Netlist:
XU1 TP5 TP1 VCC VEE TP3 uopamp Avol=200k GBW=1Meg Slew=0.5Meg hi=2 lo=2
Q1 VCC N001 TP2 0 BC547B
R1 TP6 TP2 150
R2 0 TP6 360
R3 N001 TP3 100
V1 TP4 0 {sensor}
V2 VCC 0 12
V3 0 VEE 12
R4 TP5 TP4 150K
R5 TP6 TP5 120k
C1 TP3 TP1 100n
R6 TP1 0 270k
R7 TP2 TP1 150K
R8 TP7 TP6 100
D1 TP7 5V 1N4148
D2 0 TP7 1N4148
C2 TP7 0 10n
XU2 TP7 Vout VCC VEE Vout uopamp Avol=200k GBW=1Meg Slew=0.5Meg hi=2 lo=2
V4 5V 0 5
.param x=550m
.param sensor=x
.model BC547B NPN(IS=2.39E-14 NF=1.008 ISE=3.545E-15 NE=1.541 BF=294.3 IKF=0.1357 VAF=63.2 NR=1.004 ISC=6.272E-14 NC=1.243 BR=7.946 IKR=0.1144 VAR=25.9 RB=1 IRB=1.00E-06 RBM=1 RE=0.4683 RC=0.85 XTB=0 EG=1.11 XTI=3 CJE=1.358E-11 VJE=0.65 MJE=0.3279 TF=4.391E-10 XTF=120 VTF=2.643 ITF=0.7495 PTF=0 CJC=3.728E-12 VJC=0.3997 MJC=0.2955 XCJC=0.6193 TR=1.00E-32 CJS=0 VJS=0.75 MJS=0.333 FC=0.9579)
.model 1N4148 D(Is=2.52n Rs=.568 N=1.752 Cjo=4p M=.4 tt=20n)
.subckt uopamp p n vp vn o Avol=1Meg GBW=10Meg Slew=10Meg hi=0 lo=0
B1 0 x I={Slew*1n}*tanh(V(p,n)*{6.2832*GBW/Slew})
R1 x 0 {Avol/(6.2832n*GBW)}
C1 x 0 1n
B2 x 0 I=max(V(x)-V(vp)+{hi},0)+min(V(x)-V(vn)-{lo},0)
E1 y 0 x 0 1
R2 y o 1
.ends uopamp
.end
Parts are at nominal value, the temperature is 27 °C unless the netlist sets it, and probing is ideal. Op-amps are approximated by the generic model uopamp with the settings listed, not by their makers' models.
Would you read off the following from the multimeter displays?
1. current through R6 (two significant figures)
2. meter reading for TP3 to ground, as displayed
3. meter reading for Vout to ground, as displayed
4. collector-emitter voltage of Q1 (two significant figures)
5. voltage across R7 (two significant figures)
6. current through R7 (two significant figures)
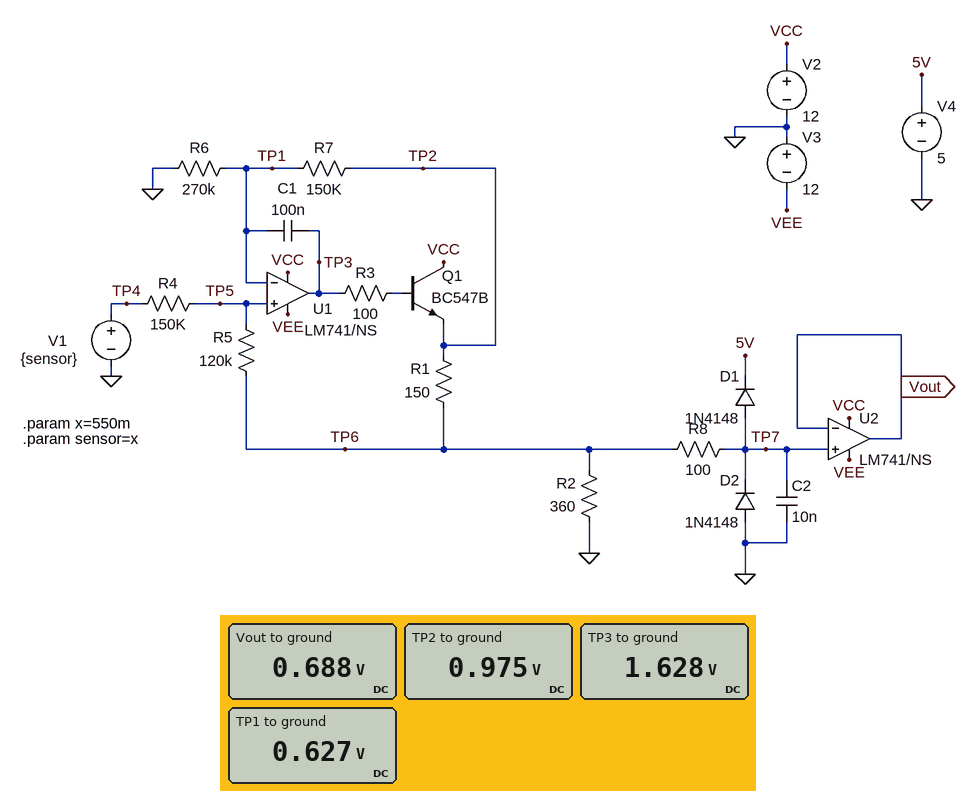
2.3 µA
1.628 V
0.688 V
11 V
350 mV
2.3 µA
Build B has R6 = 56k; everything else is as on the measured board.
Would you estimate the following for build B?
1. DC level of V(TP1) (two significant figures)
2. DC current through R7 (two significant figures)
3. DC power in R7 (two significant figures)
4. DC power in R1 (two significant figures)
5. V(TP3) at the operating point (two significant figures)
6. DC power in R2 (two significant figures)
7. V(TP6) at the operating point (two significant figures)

2.5 V
45 µA
300 µW
67 mW
10 V
100 mW
6.1 V
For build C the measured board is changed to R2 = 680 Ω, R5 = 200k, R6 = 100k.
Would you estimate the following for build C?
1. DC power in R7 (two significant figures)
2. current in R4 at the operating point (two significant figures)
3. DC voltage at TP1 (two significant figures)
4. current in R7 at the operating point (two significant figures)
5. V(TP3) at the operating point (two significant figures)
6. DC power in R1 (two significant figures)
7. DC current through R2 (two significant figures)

99 µW
13 µA
2.6 V
26 µA
7.1 V
9.0 mW
7.7 mA
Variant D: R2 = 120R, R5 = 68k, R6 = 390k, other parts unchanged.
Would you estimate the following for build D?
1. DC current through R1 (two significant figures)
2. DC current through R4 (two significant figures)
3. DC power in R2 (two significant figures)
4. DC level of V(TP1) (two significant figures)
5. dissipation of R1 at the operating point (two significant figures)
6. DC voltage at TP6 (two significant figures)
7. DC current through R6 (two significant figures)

1.5 mA
1.7 µA
280 µW
300 mV
350 µW
180 mV
760 nA
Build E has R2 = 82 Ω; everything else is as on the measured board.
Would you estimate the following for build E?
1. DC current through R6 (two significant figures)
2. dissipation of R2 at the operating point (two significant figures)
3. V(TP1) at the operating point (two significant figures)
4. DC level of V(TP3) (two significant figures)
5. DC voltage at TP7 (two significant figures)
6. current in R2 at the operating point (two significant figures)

1.3 µA
460 µW
350 mV
1.2 V
190 mV
2.4 mA
